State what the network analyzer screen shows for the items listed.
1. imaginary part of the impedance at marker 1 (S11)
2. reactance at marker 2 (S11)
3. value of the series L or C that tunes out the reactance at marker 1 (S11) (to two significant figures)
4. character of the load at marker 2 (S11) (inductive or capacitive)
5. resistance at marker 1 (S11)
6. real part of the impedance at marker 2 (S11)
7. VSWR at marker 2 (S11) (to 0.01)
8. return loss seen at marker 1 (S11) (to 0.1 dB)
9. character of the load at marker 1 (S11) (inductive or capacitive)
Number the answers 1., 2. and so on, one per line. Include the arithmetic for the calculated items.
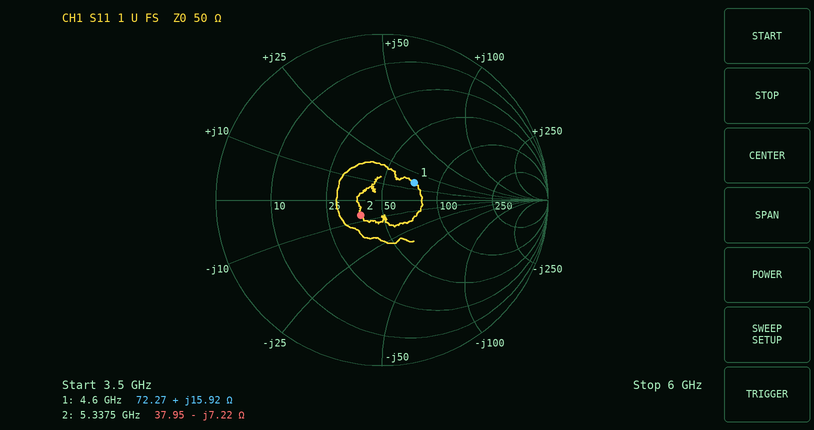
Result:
1. +15.92 Ω
2. -7.22 Ω
3. C = 1/(2π × 4.6 GHz × 15.92 Ω) ≈ 2.2 pF
4. capacitive
5. 72.27 Ω
6. 37.95 Ω
7. 1.38
8. 13.1 dB
9. inductive
